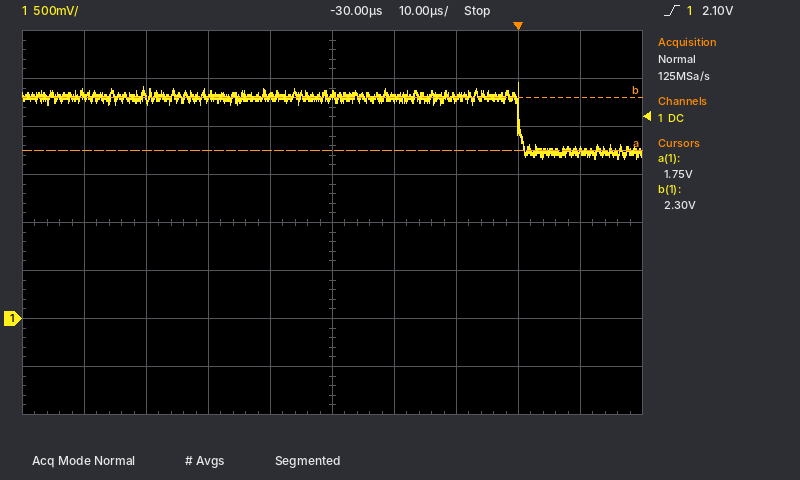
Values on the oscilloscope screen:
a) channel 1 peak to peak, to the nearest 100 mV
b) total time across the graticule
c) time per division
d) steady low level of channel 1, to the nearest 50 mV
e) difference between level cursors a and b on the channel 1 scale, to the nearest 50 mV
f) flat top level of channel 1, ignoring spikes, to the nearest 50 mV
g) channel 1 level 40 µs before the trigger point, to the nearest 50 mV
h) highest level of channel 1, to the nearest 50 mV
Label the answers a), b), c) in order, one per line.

a) 800 mV
b) 100 µs
c) 10 µs
d) 1.75 V
e) 550 mV
f) 2.30 V
g) 2.30 V
h) 2.45 V
